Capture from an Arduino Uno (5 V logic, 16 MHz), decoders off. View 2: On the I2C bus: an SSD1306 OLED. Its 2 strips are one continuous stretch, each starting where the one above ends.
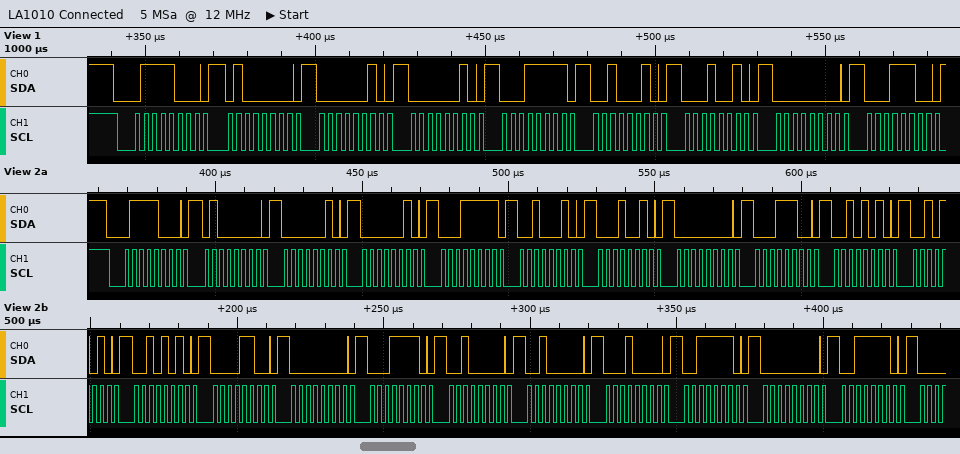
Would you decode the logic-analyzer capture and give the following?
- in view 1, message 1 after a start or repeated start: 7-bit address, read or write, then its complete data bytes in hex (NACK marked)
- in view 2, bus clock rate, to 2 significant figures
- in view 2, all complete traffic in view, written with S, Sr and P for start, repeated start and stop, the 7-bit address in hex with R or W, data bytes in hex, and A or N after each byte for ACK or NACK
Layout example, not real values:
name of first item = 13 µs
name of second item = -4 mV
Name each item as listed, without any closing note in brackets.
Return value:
in view 1, message 1 after a start or repeated start: 7-bit address, read or write, then its complete data bytes in hex = 0x3C write: 40 02 02 1F 22 12 00 1C
in view 2, bus clock rate, to 2 significant figures = 400 kHz
in view 2, all complete traffic in view, written with S, Sr and P for start, repeated start and stop, the 7-bit address in hex with R or W, data bytes in hex, and A or N after each byte for ACK or NACK = S 3CW A 40 A 02 A 02 A 1F A 22 A 12 A 00 A 1C A 2A A 2A A 2A A 0C A 00 A 1E A 20 A 20 A 10 A 3E A 00 A 3E A
